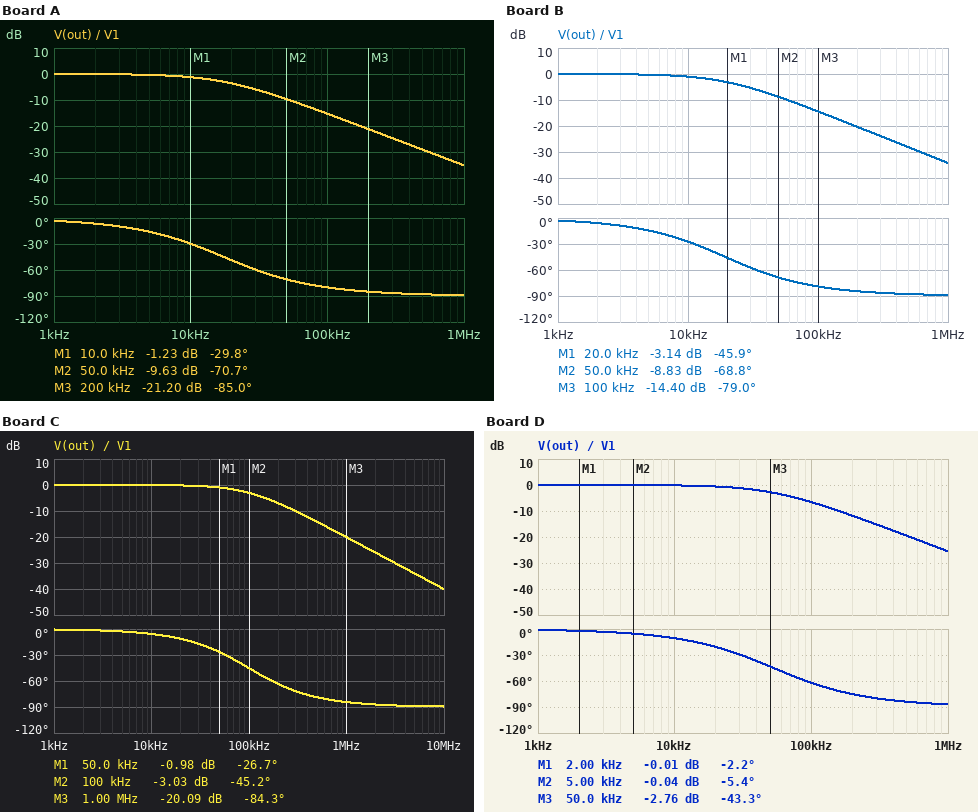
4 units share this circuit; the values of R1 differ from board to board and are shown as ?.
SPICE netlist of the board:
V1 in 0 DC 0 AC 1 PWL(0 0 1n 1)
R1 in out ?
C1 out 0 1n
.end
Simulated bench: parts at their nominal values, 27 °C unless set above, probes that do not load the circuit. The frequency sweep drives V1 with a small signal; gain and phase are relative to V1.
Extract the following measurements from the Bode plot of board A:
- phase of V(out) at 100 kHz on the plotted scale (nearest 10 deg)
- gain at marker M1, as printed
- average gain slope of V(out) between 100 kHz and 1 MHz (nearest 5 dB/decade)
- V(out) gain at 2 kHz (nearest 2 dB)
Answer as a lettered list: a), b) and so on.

a) -80 deg
b) -1.23 dB
c) -20 dB/decade
d) 0 dB
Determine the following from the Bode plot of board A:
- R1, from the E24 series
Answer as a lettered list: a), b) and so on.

a) 9.1 kΩ
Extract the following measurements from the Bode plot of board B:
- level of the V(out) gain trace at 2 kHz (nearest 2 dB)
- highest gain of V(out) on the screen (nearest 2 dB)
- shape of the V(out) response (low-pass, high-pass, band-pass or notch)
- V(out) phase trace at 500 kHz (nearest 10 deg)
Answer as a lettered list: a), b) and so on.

a) 0 dB
b) 0 dB
c) low-pass
d) -90 deg
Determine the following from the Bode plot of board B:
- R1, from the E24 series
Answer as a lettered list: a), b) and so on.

a) 8.2 kΩ
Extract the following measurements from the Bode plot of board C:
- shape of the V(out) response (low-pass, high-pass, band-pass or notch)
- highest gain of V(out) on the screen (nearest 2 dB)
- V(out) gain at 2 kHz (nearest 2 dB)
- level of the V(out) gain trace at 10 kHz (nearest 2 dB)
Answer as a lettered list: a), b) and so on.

a) low-pass
b) 0 dB
c) 0 dB
d) 0 dB
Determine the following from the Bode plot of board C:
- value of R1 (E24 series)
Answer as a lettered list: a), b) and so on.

a) 1.6 kΩ
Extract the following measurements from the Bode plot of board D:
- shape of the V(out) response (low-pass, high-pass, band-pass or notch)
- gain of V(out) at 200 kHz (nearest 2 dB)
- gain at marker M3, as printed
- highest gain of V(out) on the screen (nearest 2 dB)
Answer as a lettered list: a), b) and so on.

a) low-pass
b) -12 dB
c) -2.76 dB
d) 0 dB
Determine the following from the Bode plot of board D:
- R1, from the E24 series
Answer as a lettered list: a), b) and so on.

a) 3 kΩ
